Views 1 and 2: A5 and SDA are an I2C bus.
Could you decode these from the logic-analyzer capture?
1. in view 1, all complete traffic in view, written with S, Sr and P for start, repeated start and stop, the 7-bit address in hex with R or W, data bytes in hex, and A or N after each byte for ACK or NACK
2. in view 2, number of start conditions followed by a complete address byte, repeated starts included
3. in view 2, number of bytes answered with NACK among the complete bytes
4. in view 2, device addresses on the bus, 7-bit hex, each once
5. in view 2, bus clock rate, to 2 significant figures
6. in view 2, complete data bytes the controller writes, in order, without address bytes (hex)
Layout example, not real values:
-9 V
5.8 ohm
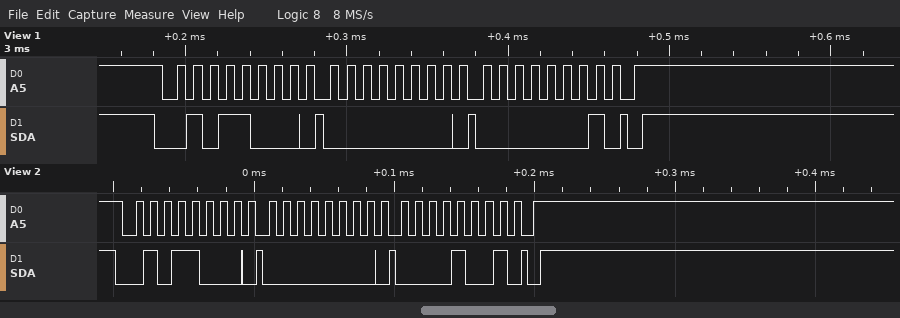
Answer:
S 2CW A 00 A 01 A P
1
0
0x2C
100 kHz
00 09
